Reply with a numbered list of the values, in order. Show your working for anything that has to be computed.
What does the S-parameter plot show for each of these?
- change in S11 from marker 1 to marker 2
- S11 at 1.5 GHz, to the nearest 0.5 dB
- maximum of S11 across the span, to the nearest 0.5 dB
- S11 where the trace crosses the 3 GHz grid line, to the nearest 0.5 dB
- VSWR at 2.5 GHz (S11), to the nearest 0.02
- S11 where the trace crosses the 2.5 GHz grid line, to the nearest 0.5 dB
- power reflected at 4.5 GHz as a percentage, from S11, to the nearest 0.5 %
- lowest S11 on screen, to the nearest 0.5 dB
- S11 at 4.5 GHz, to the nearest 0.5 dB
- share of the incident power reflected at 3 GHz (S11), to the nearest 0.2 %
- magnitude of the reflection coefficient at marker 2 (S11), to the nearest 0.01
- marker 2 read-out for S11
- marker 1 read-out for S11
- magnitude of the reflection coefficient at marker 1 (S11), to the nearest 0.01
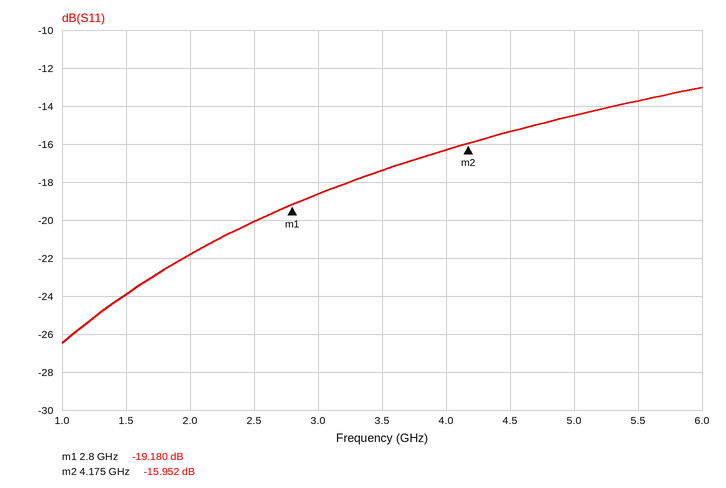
1. -15.952 − (-19.18) = 3.228 dB
2. -24.0 dB
3. -13.0 dB
4. -18.5 dB
5. |Γ| = 10^(-20/20) = 0.1000; VSWR = (1 + 0.1000)/(1 − 0.1000) ≈ 1.22
6. -20.0 dB
7. 10^(-15.5/10) ≈ 2.82 %, so 3.0 % to the nearest 0.5 %
8. -26.5 dB
9. -15.5 dB
10. 10^(-18.5/10) ≈ 1.4 %
11. 10^(-15.952/20) ≈ 0.16
12. -15.952 dB
13. -19.180 dB
14. 10^(-19.18/20) ≈ 0.11
